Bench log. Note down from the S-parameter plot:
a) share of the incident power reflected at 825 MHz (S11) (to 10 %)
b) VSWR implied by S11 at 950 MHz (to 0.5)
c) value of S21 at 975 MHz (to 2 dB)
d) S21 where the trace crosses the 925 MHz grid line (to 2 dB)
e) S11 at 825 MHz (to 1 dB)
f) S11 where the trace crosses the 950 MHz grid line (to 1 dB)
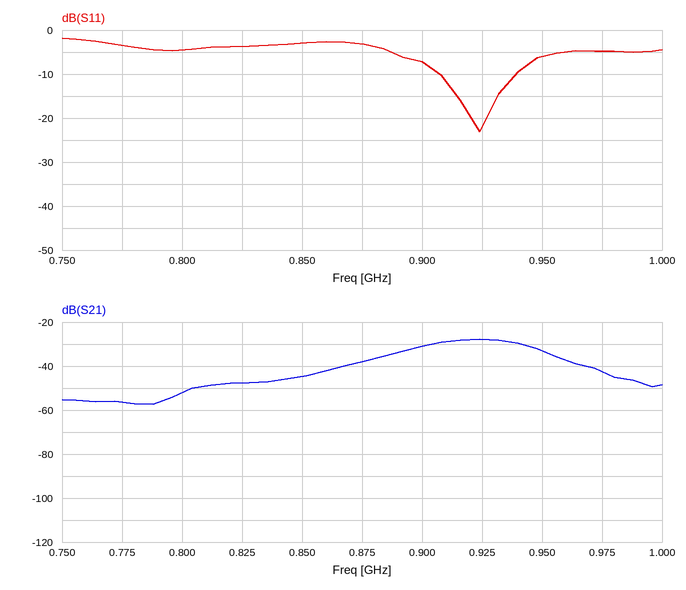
40 %
3.0
-42 dB
-28 dB
-4 dB
-6 dB
